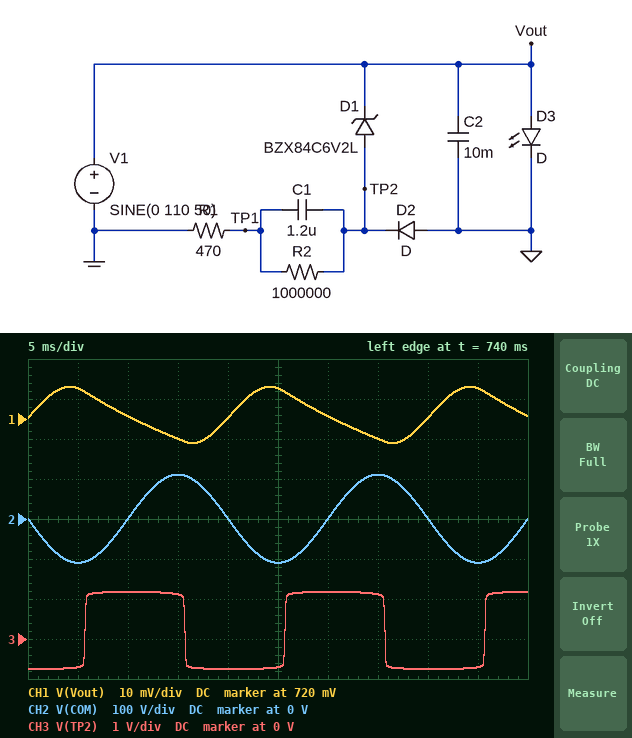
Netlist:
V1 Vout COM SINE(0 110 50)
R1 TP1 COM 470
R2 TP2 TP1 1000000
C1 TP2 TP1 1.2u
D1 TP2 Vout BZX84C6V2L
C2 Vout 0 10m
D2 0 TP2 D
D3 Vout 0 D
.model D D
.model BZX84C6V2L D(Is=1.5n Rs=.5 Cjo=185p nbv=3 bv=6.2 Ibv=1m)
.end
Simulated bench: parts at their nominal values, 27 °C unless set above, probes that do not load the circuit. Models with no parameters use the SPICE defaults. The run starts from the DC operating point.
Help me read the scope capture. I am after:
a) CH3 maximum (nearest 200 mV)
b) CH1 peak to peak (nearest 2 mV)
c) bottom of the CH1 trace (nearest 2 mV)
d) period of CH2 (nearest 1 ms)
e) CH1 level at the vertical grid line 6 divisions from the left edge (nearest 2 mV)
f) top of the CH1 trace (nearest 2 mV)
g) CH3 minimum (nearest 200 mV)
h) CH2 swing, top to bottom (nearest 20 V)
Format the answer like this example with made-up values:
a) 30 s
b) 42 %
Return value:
a) 1.2 V
b) 14 mV
c) 714 mV
d) 20 ms
e) 720 mV
f) 728 mV
g) -800 mV
h) 220 V
